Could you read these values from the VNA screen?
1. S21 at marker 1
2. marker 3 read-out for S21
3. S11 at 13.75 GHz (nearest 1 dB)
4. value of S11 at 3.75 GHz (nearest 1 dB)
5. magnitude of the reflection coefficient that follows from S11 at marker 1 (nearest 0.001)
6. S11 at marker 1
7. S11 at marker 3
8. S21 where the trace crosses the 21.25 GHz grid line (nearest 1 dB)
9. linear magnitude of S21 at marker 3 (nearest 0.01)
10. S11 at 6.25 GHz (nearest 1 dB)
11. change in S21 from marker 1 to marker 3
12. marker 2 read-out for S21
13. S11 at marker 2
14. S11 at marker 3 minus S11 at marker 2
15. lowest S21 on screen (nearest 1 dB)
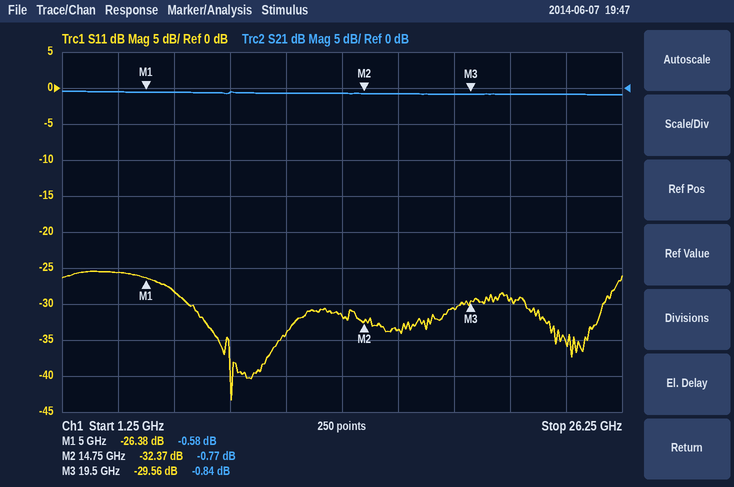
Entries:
-0.58 dB
-0.84 dB
-32 dB
-26 dB
0.048
-26.38 dB
-29.56 dB
-1 dB
0.91
-28 dB
-0.26 dB
-0.77 dB
-32.37 dB
2.81 dB
-1 dB
